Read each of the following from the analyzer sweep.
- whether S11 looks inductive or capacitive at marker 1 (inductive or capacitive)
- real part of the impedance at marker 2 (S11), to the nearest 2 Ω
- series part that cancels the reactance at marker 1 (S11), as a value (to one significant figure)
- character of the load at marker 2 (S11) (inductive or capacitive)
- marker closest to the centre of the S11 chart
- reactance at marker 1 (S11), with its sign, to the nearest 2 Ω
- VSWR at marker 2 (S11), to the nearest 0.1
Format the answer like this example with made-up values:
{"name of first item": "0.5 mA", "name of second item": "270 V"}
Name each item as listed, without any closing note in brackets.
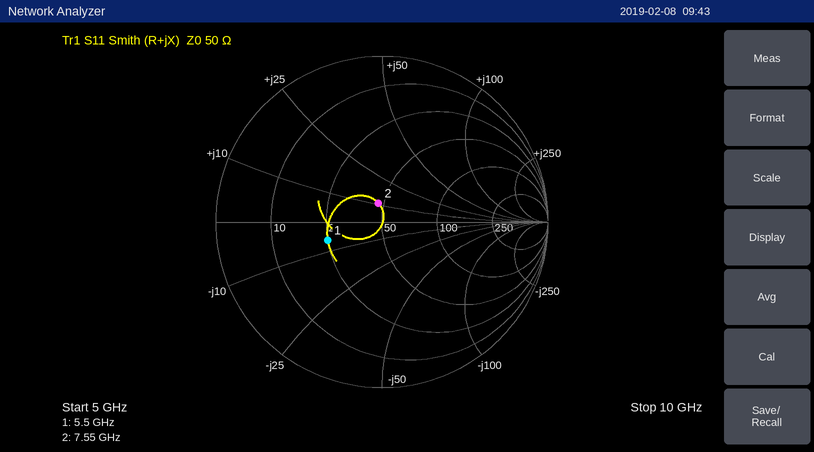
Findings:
{"whether S11 looks inductive or capacitive at marker 1": "capacitive", "real part of the impedance at marker 2 (S11), to the nearest 2 Ω": "46 Ω", "series part that cancels the reactance at marker 1 (S11), as a value": "200 pH", "character of the load at marker 2 (S11)": "inductive", "marker closest to the centre of the S11 chart": "marker 2", "reactance at marker 1 (S11), with its sign, to the nearest 2 Ω": "-6 Ω", "VSWR at marker 2 (S11), to the nearest 0.1": "1.3"}
